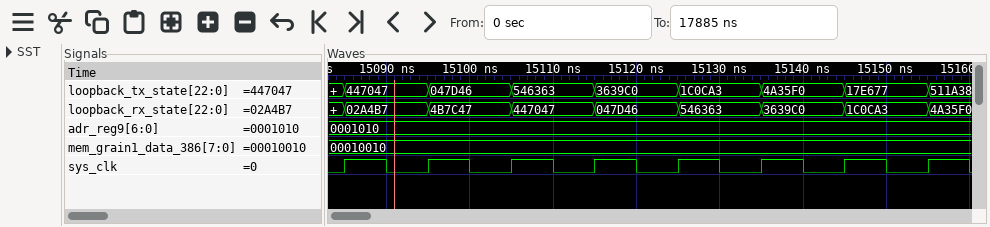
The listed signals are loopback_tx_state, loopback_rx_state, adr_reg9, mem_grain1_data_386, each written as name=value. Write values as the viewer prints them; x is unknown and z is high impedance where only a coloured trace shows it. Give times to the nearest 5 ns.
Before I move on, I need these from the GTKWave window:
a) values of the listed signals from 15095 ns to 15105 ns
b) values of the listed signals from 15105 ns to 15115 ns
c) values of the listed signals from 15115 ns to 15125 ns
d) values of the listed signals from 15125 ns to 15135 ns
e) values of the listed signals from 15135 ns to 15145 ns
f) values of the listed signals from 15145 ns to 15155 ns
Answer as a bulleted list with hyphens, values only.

- loopback_tx_state=047D46, loopback_rx_state=4B7C47, adr_reg9=0001010, mem_grain1_data_386=00010010
- loopback_tx_state=546363, loopback_rx_state=447047, adr_reg9=0001010, mem_grain1_data_386=00010010
- loopback_tx_state=3639C0, loopback_rx_state=047D46, adr_reg9=0001010, mem_grain1_data_386=00010010
- loopback_tx_state=1C0CA3, loopback_rx_state=546363, adr_reg9=0001010, mem_grain1_data_386=00010010
- loopback_tx_state=4A35F0, loopback_rx_state=3639C0, adr_reg9=0001010, mem_grain1_data_386=00010010
- loopback_tx_state=17E677, loopback_rx_state=1C0CA3, adr_reg9=0001010, mem_grain1_data_386=00010010
